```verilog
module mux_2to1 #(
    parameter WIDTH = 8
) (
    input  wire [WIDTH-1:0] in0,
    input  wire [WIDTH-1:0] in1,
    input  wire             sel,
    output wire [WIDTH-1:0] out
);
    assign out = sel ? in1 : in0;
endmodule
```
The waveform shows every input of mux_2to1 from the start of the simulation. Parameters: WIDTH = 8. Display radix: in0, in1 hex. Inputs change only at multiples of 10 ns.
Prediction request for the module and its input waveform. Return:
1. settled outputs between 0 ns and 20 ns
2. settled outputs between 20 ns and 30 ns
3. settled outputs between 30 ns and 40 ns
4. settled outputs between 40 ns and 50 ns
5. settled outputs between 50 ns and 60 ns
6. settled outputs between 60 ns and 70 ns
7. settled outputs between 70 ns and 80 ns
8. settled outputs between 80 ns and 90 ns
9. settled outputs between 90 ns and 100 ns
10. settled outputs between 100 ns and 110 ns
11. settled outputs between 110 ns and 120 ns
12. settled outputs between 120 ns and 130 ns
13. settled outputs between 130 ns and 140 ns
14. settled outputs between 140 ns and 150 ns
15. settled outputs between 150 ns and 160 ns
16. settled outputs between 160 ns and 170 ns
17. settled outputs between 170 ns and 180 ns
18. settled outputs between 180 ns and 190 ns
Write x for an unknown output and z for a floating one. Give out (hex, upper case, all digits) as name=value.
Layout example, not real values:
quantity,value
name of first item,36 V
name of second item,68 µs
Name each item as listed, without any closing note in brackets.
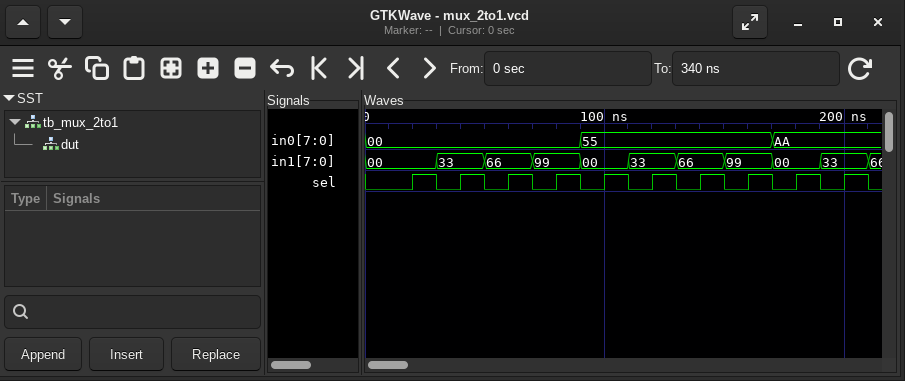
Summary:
quantity,value
settled outputs between 0 ns and 20 ns,out=00
settled outputs between 20 ns and 30 ns,out=00
settled outputs between 30 ns and 40 ns,out=00
settled outputs between 40 ns and 50 ns,out=33
settled outputs between 50 ns and 60 ns,out=00
settled outputs between 60 ns and 70 ns,out=66
settled outputs between 70 ns and 80 ns,out=00
settled outputs between 80 ns and 90 ns,out=99
settled outputs between 90 ns and 100 ns,out=55
settled outputs between 100 ns and 110 ns,out=00
settled outputs between 110 ns and 120 ns,out=55
settled outputs between 120 ns and 130 ns,out=33
settled outputs between 130 ns and 140 ns,out=55
settled outputs between 140 ns and 150 ns,out=66
settled outputs between 150 ns and 160 ns,out=55
settled outputs between 160 ns and 170 ns,out=99
settled outputs between 170 ns and 180 ns,out=AA
settled outputs between 180 ns and 190 ns,out=00
